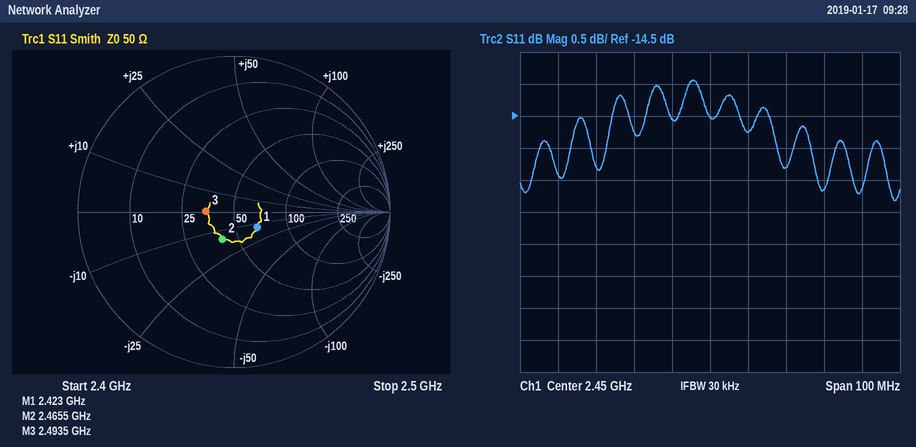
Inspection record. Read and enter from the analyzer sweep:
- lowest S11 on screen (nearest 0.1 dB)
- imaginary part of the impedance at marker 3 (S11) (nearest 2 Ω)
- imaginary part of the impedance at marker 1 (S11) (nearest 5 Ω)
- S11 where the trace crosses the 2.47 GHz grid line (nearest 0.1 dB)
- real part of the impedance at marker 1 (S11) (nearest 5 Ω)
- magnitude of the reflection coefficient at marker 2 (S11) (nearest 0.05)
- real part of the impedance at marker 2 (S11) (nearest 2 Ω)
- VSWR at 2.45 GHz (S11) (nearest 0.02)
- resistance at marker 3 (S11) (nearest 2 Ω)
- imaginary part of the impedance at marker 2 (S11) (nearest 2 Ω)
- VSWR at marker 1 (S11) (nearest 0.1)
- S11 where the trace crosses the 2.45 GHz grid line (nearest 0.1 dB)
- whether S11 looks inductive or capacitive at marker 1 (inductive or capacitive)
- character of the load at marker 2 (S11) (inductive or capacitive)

-15.8 dB
0 Ω
-15 Ω
-15.3 dB
65 Ω
0.20
40 Ω
1.46
34 Ω
-14 Ω
1.4
-14.5 dB
capacitive
capacitive
